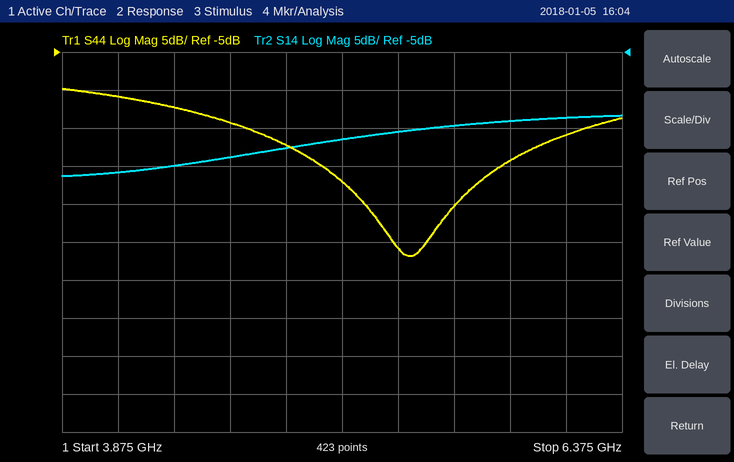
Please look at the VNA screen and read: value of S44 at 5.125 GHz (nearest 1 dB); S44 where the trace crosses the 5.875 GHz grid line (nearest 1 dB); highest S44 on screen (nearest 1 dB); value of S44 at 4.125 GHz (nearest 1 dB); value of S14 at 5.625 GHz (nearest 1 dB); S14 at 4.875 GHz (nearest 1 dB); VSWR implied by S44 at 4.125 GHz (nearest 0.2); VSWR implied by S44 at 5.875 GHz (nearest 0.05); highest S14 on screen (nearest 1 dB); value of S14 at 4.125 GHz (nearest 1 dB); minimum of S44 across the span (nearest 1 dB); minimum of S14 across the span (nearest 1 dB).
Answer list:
-22 dB
-19 dB
-10 dB
-11 dB
-15 dB
-18 dB
1.8
1.25
-13 dB
-21 dB
-32 dB
-21 dB
